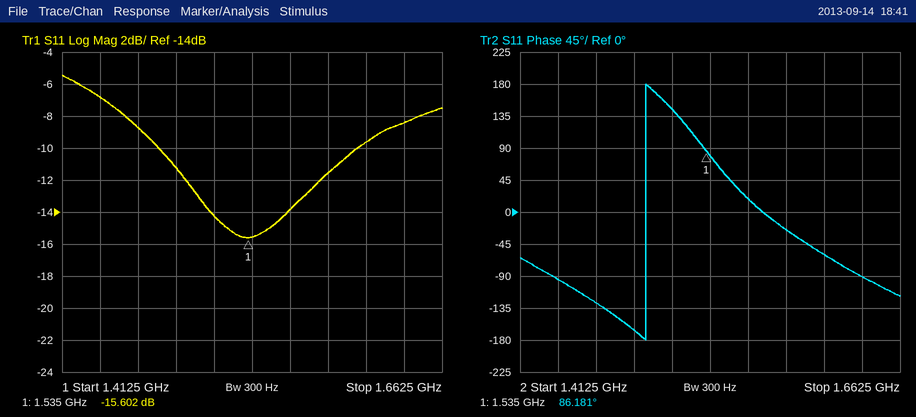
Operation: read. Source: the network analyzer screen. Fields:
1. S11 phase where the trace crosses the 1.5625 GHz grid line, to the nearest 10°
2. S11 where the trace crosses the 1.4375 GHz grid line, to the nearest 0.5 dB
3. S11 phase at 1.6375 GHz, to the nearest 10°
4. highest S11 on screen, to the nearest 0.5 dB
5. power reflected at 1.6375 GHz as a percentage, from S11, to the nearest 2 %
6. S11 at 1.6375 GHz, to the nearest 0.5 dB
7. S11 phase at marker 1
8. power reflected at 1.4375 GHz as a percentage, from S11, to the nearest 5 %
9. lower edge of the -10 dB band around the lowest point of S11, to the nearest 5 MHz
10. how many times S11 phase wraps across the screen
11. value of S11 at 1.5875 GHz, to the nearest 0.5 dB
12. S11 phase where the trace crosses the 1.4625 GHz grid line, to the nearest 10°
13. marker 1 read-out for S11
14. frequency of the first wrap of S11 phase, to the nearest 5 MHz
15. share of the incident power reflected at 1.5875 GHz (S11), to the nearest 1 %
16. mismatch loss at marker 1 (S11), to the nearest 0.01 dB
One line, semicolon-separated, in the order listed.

20°; -7.0 dB; -90°; -5.5 dB; 14 %; -8.5 dB; 86.181°; 20 %; 1.475 GHz; 1; -11.5 dB; -130°; -15.602 dB; 1.495 GHz; 7 %; 0.12 dB
